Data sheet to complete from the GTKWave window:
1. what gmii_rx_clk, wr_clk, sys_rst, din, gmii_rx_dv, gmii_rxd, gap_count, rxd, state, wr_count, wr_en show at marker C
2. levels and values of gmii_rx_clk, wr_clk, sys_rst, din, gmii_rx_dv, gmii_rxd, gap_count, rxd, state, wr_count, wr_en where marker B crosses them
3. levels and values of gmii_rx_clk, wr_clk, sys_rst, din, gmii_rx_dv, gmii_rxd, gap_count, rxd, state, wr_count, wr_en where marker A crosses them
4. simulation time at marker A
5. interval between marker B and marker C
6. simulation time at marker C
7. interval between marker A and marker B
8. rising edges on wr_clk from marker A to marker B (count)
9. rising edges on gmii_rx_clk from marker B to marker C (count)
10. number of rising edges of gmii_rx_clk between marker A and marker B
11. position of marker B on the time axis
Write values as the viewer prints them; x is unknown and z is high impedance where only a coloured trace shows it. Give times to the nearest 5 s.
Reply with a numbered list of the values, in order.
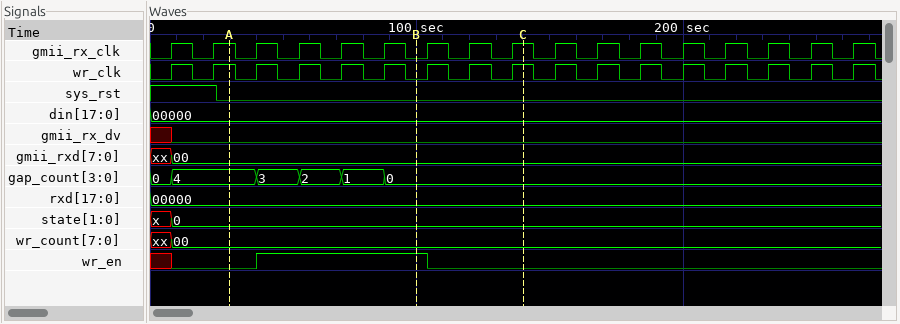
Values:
1. gmii_rx_clk=1, wr_clk=1, sys_rst=0, din=00000, gmii_rx_dv=0, gmii_rxd=00, gap_count=0, rxd=00000, state=0, wr_count=00, wr_en=0
2. gmii_rx_clk=0, wr_clk=0, sys_rst=0, din=00000, gmii_rx_dv=0, gmii_rxd=00, gap_count=0, rxd=00000, state=0, wr_count=00, wr_en=1
3. gmii_rx_clk=1, wr_clk=1, sys_rst=0, din=00000, gmii_rx_dv=0, gmii_rxd=00, gap_count=4, rxd=00000, state=0, wr_count=00, wr_en=0
4. 30 s
5. 40 s
6. 140 s
7. 70 s
8. 4
9. 3
10. 4
11. 100 s
